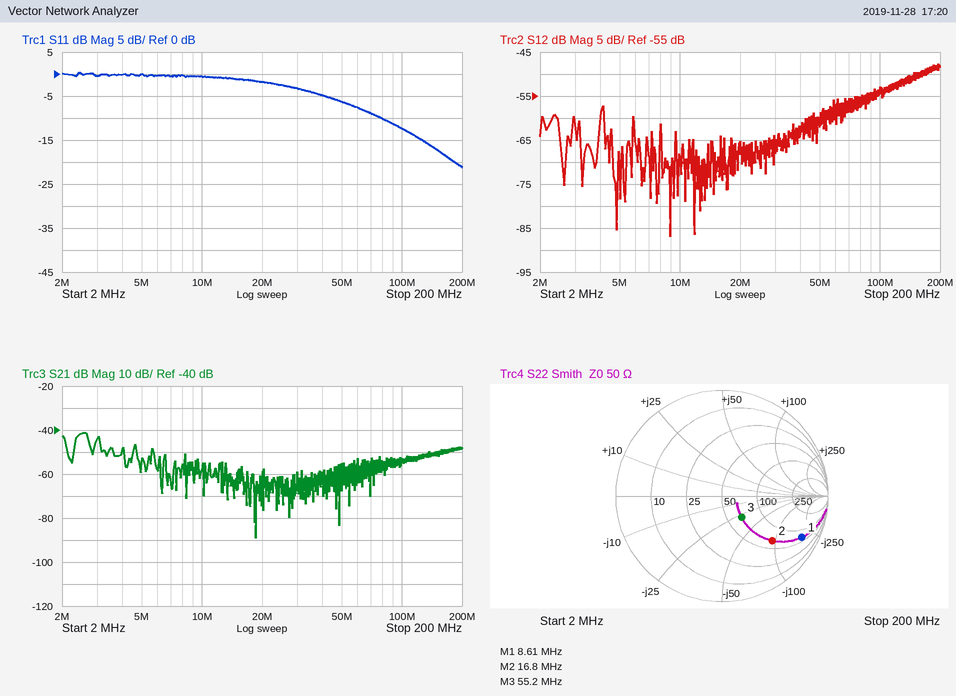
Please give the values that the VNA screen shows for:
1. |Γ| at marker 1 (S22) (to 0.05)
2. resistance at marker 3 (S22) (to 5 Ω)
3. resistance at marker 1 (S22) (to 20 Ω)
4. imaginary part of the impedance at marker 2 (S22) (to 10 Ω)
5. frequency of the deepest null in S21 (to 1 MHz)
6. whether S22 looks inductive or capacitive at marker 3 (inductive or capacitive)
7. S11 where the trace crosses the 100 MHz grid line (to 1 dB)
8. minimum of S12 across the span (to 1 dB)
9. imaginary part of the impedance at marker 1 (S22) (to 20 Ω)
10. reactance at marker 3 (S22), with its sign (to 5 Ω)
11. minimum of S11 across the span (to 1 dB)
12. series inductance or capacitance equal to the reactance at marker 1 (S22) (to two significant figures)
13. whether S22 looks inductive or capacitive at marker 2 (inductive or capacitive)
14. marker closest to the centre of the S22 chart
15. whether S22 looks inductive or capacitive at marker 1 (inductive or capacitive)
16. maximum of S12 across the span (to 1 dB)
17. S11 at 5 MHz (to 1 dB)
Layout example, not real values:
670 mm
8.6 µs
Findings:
0.85
65 Ω
60 Ω
-90 Ω
19 MHz
capacitive
-12 dB
-87 dB
-180 Ω
-30 Ω
-21 dB
100 pF
capacitive
marker 3
capacitive
-48 dB
0 dB
